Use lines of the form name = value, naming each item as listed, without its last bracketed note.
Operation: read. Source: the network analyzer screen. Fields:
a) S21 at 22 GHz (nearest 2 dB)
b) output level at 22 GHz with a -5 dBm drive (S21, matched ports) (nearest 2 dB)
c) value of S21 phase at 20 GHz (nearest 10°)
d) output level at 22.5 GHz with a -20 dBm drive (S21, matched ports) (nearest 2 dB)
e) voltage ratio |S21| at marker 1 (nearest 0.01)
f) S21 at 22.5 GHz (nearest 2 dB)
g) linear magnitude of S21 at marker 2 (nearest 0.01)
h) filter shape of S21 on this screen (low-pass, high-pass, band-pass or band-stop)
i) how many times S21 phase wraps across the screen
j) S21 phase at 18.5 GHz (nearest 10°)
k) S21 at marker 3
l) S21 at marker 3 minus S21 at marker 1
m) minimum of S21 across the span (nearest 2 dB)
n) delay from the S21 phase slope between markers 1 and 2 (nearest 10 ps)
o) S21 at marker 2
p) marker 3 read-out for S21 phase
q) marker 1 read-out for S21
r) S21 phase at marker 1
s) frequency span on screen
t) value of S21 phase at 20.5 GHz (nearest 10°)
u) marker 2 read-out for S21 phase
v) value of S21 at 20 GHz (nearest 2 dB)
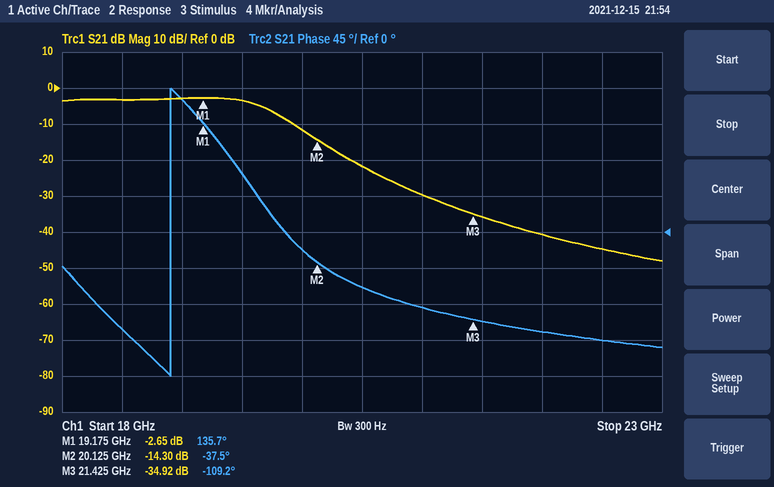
S21 at 22 GHz = -40 dB
output level at 22 GHz with a -5 dBm drive (S21, matched ports) = -46 dBm
value of S21 phase at 20 GHz = -20°
output level at 22.5 GHz with a -20 dBm drive (S21, matched ports) = -64 dBm
voltage ratio |S21| at marker 1 = 0.74
S21 at 22.5 GHz = -44 dB
linear magnitude of S21 at marker 2 = 0.19
filter shape of S21 on this screen = low-pass
how many times S21 phase wraps across the screen = 1
S21 phase at 18.5 GHz = -120°
S21 at marker 3 = -34.92 dB
S21 at marker 3 minus S21 at marker 1 = -32.27 dB
minimum of S21 across the span = -48 dB
delay from the S21 phase slope between markers 1 and 2 = 510 ps
S21 at marker 2 = -14.30 dB
marker 3 read-out for S21 phase = -109.2°
marker 1 read-out for S21 = -2.65 dB
S21 phase at marker 1 = 135.7°
frequency span on screen = 5 GHz
value of S21 phase at 20.5 GHz = -70°
marker 2 read-out for S21 phase = -37.5°
value of S21 at 20 GHz = -12 dB
